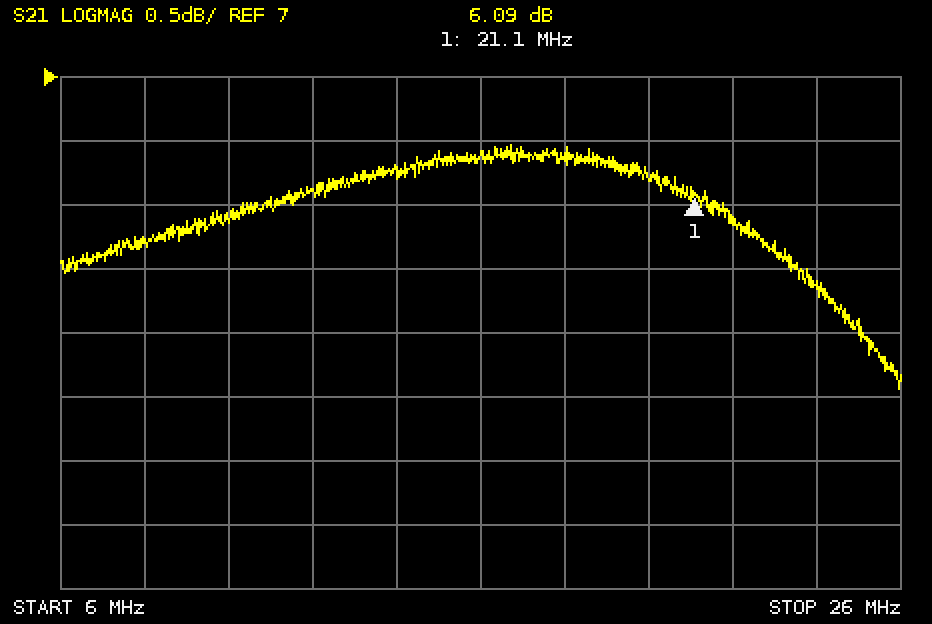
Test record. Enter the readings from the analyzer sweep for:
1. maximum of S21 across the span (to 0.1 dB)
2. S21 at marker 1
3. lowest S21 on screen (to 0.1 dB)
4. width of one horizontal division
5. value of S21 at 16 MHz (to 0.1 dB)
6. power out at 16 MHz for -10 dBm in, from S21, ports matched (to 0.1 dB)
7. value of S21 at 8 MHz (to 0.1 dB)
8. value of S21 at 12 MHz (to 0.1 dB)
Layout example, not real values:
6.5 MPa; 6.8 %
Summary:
6.5 dB; 6.09 dB; 4.6 dB; 2 MHz; 6.4 dB; -3.6 dBm; 5.7 dB; 6.1 dB
